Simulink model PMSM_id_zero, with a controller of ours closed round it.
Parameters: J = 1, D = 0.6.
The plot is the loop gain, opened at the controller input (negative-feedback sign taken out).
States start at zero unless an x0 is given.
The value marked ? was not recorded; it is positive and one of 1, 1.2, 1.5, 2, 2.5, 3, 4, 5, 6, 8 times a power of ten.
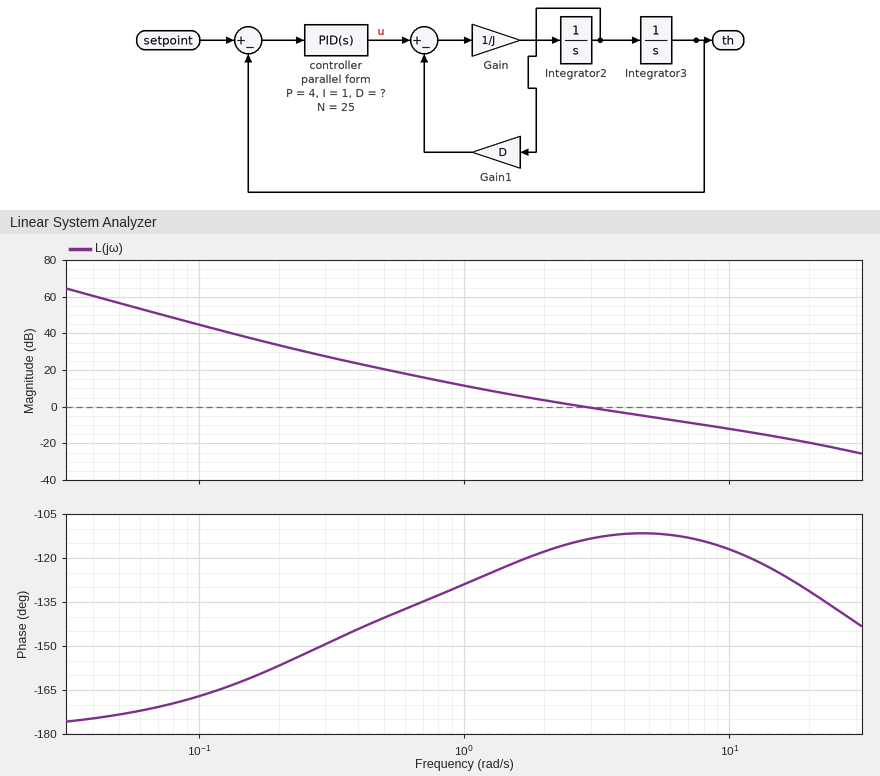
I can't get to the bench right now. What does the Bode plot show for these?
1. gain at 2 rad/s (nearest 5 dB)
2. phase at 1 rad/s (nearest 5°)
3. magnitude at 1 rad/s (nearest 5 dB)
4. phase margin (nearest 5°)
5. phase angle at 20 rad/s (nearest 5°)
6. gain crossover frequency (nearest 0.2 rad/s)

5 dB
-130°
10 dB
65°
-130°
2.8 rad/s
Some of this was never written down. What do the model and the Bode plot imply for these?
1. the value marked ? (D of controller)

2.5
